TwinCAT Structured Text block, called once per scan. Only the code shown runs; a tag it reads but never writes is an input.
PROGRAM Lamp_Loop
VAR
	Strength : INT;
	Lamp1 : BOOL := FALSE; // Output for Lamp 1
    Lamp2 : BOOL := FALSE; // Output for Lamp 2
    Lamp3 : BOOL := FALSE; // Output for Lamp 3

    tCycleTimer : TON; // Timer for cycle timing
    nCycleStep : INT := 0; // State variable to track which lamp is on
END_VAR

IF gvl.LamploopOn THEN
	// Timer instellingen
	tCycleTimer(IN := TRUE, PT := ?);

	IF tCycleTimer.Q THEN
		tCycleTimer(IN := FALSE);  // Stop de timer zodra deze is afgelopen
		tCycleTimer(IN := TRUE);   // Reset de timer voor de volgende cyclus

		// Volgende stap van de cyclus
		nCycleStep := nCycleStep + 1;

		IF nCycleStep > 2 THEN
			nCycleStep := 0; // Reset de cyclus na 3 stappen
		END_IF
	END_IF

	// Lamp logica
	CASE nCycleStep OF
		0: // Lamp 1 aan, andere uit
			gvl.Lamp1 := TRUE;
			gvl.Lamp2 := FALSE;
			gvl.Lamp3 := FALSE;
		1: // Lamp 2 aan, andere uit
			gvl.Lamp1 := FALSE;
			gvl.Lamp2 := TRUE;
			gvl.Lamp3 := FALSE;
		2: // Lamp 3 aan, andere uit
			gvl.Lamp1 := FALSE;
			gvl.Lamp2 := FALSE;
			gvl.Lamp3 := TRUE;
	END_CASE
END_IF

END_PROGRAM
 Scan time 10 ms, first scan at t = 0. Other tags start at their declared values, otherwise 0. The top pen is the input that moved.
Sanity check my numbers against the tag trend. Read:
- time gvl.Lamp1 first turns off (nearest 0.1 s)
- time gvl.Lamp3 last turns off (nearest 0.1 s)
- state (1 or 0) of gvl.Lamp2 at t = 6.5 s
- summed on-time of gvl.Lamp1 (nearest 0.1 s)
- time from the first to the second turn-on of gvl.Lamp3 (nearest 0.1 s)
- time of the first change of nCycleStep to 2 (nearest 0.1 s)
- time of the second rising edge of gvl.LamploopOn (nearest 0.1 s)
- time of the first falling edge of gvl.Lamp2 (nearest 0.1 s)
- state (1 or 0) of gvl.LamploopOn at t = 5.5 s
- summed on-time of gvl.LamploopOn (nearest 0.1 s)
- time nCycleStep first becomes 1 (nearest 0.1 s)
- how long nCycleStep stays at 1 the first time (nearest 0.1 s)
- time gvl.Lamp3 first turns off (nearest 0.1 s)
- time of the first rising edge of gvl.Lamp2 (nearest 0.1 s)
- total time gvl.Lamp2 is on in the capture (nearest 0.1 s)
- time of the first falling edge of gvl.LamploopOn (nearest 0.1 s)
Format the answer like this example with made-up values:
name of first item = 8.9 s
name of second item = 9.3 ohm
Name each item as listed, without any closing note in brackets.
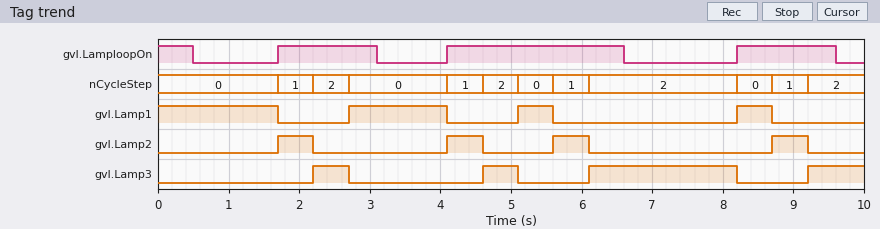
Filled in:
time gvl.Lamp1 first turns off = 1.7 s
time gvl.Lamp3 last turns off = 8.2 s
state (1 or 0) of gvl.Lamp2 at t = 6.5 s = 0
summed on-time of gvl.Lamp1 = 4.1 s
time from the first to the second turn-on of gvl.Lamp3 = 2.4 s
time of the first change of nCycleStep to 2 = 2.2 s
time of the second rising edge of gvl.LamploopOn = 4.1 s
time of the first falling edge of gvl.Lamp2 = 2.2 s
state (1 or 0) of gvl.LamploopOn at t = 5.5 s = 1
summed on-time of gvl.LamploopOn = 5.8 s
time nCycleStep first becomes 1 = 1.7 s
how long nCycleStep stays at 1 the first time = 0.5 s
time gvl.Lamp3 first turns off = 2.7 s
time of the first rising edge of gvl.Lamp2 = 1.7 s
total time gvl.Lamp2 is on in the capture = 2.0 s
time of the first falling edge of gvl.LamploopOn = 0.5 s
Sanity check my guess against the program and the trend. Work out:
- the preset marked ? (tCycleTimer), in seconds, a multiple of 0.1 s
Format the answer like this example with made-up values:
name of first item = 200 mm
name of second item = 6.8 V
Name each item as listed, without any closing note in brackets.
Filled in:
the preset marked ? (tCycleTimer), in seconds, a multiple of 0.1 s = 0.5 s
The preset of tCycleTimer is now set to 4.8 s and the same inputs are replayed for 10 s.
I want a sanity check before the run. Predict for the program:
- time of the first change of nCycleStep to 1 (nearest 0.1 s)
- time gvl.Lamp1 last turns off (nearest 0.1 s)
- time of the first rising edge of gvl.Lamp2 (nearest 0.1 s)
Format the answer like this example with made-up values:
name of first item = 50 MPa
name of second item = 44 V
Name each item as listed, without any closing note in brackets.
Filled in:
time of the first change of nCycleStep to 1 = 4.8 s
time gvl.Lamp1 last turns off = 4.8 s
time of the first rising edge of gvl.Lamp2 = 4.8 s
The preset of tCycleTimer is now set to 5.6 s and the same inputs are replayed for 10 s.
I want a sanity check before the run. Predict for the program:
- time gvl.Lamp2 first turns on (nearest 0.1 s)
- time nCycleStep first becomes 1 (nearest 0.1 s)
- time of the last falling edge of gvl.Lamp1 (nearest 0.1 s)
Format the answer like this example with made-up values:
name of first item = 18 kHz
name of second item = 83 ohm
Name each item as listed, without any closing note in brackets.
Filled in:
time gvl.Lamp2 first turns on = 5.6 s
time nCycleStep first becomes 1 = 5.6 s
time of the last falling edge of gvl.Lamp1 = 5.6 s
